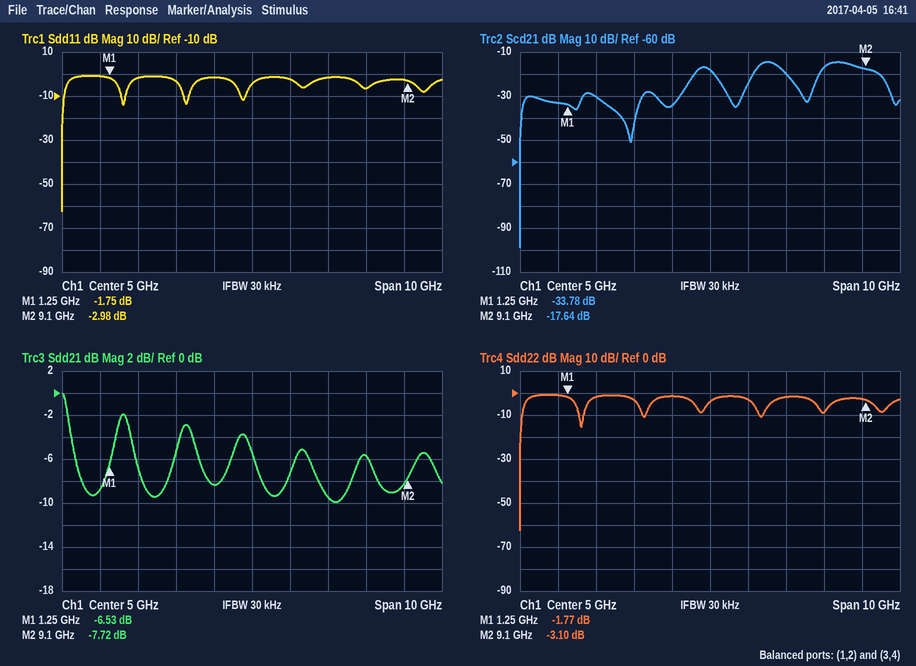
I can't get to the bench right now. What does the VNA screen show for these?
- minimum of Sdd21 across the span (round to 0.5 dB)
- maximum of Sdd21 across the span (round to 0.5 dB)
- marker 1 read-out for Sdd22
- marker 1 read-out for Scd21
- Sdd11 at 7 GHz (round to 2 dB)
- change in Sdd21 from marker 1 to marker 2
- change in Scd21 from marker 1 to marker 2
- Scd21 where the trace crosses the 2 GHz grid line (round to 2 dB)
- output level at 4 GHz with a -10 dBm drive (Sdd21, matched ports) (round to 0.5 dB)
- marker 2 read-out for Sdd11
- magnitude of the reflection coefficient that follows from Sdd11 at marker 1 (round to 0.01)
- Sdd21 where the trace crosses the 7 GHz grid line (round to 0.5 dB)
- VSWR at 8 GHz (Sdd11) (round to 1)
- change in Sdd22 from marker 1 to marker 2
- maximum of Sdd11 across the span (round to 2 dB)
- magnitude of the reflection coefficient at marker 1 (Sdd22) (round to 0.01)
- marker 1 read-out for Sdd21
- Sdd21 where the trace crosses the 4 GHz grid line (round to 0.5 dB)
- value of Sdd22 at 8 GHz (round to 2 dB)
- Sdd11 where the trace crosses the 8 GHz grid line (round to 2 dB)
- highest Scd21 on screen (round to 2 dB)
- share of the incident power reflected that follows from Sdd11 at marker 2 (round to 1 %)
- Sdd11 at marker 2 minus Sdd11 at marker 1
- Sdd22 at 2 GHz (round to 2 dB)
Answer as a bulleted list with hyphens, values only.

- -10.0 dB
- 0.0 dB
- -1.77 dB
- -33.78 dB
- -2 dB
- -1.19 dB
- 16.14 dB
- -30 dB
- -18.5 dBm
- -2.98 dB
- 0.82
- -9.5 dB
- 3
- -1.33 dB
- 0 dB
- 0.82
- -6.53 dB
- -8.5 dB
- -8 dB
- -6 dB
- -14 dB
- 50 %
- -1.23 dB
- -2 dB
